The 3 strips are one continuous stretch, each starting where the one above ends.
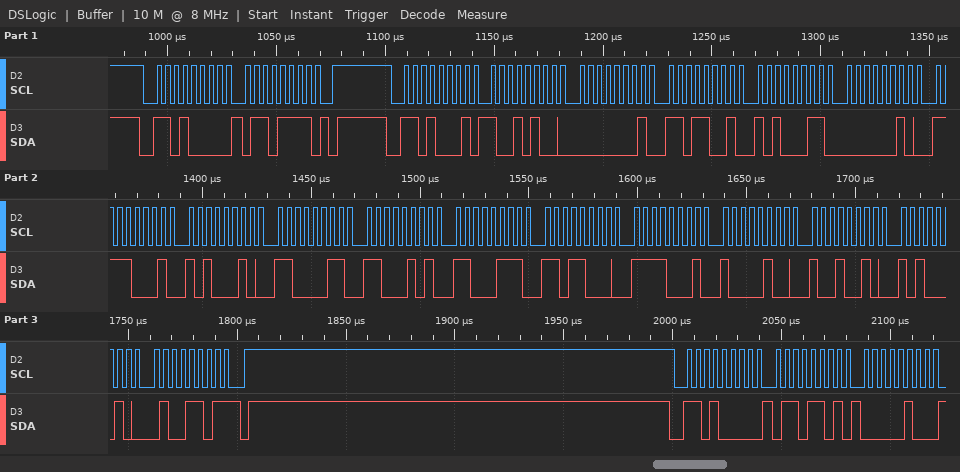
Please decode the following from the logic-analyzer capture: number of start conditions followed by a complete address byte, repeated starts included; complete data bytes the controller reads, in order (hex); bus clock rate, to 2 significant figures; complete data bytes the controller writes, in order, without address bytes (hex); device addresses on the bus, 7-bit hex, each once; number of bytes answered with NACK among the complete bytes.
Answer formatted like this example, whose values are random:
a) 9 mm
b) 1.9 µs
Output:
a) 3
b) 94 01 D9 A3 02 F1 A2 C3 C5 C7 D8 F1 84 92 A2 4D
c) 250 kHz
d) 6F 6D 04
e) 0x68
f) 1
